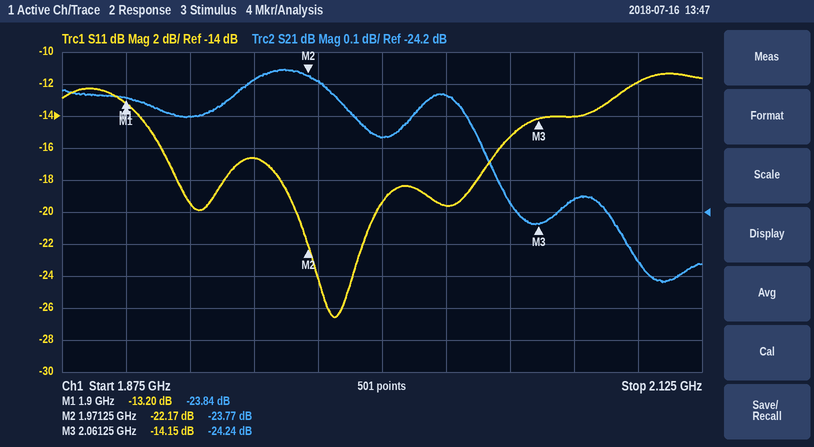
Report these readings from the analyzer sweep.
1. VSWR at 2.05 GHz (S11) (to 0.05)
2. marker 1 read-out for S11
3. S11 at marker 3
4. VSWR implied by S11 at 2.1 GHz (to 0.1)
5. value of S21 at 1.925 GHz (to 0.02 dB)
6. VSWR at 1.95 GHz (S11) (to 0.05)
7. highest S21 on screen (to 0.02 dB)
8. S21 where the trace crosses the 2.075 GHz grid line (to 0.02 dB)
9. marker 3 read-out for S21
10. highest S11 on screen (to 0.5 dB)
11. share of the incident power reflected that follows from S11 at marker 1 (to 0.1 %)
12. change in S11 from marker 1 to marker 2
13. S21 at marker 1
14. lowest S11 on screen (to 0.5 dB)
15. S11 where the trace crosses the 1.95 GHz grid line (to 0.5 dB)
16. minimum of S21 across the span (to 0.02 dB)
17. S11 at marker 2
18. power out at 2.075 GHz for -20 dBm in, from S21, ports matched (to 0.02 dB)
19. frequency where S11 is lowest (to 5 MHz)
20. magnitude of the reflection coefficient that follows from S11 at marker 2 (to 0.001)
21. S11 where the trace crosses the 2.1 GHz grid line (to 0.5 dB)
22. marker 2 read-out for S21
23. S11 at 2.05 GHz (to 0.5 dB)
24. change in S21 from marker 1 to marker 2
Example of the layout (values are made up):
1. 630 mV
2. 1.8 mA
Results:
1. 1.40
2. -13.20 dB
3. -14.15 dB
4. 1.7
5. -23.90 dB
6. 1.35
7. -23.76 dB
8. -24.16 dB
9. -24.24 dB
10. -11.5 dB
11. 4.8 %
12. -8.97 dB
13. -23.84 dB
14. -26.5 dB
15. -16.5 dB
16. -24.42 dB
17. -22.17 dB
18. -44.16 dBm
19. 1.980 GHz
20. 0.078
21. -12.0 dB
22. -23.77 dB
23. -15.5 dB
24. 0.07 dB
